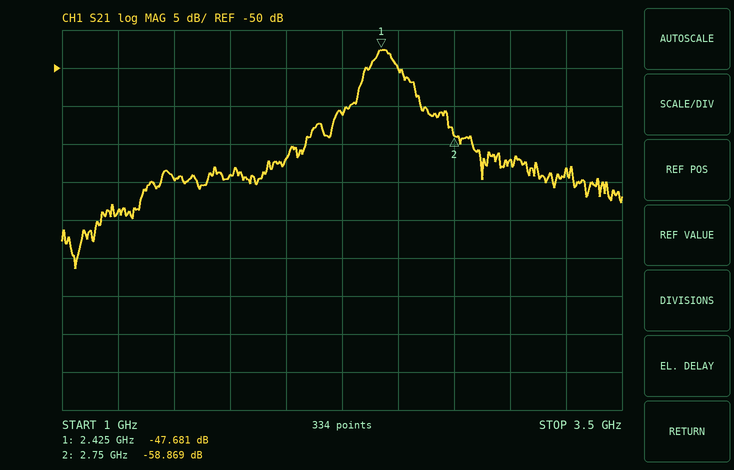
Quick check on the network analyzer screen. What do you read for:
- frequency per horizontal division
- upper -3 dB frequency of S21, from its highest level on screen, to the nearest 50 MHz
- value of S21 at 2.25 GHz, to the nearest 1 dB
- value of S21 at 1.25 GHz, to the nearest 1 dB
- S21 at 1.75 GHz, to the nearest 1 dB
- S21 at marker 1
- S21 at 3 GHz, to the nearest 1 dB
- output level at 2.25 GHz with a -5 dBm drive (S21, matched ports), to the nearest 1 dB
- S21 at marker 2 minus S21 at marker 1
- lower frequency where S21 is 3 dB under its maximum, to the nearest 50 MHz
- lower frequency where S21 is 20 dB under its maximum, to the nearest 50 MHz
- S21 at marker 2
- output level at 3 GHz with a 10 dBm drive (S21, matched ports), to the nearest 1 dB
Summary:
250 MHz
2.50 GHz
-56 dB
-69 dB
-64 dB
-47.681 dB
-62 dB
-61 dBm
-11.188 dB
2.35 GHz
1.35 GHz
-58.869 dB
-52 dBm
